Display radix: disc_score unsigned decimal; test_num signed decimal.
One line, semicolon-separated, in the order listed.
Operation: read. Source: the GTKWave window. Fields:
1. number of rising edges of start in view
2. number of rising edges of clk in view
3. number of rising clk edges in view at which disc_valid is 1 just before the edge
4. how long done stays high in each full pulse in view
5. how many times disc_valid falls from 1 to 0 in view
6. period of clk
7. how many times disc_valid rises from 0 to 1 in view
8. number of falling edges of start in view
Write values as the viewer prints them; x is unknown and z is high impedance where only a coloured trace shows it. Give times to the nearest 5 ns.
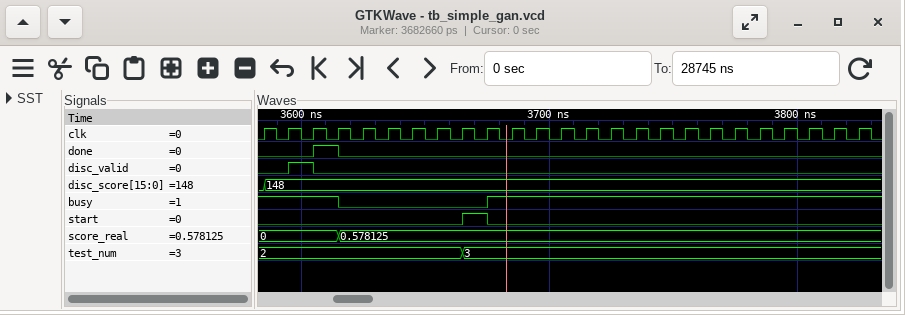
1; 25; 1; 10 ns; 1; 10 ns; 1; 1
